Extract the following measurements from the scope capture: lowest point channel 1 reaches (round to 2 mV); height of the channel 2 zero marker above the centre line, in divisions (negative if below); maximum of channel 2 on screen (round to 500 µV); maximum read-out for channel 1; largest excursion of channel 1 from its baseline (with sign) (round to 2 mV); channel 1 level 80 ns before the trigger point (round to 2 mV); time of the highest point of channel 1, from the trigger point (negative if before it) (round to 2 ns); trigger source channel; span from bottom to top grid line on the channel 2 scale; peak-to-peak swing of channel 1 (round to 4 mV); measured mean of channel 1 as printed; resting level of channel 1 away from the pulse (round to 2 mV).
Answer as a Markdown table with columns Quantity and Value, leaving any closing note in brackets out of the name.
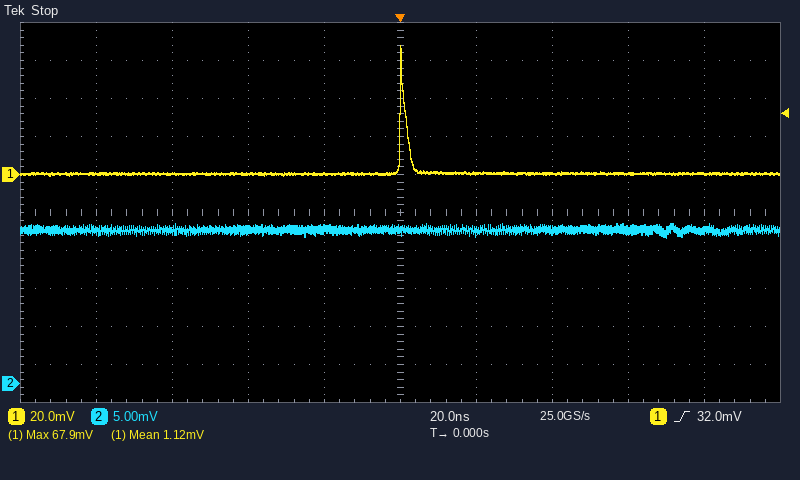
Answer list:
| Quantity | Value |
|---|---|
| lowest point channel 1 reaches | 0 mV |
| height of the channel 2 zero marker above the centre line, in divisions | -4.5 div |
| maximum of channel 2 on screen | 21.0 mV |
| maximum read-out for channel 1 | 67.9 mV |
| largest excursion of channel 1 from its baseline (with sign) | +68 mV |
| channel 1 level 80 ns before the trigger point | 0 mV |
| time of the highest point of channel 1, from the trigger point (negative if before it) | 0 ns |
| trigger source channel | channel 1 |
| span from bottom to top grid line on the channel 2 scale | 50 mV |
| peak-to-peak swing of channel 1 | 68 mV |
| measured mean of channel 1 as printed | 1.12 mV |
| resting level of channel 1 away from the pulse | 0 mV |
